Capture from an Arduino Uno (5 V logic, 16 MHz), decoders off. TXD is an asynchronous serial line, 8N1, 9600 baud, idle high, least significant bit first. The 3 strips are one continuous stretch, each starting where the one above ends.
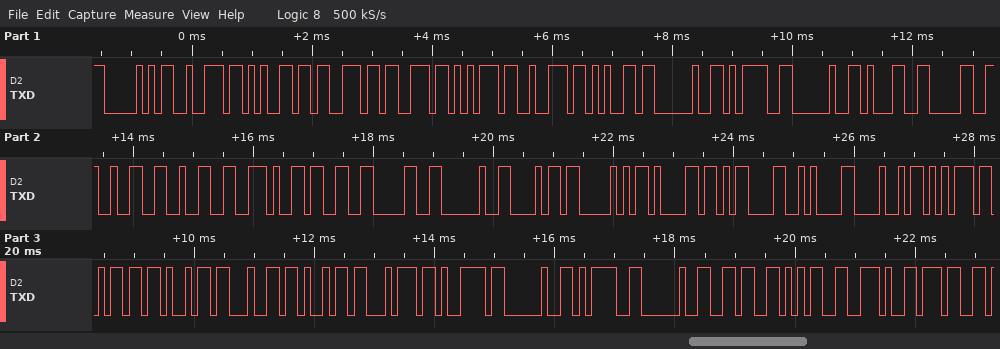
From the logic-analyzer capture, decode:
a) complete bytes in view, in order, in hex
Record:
50 72 65 73 73 75 72 65 20 3D 20 31 30 32 32 2E 33 30 20 68 50 61 0D 0A 48 75 6D 69 64 69 74 79 20 3D 20 36 35 2E 37
